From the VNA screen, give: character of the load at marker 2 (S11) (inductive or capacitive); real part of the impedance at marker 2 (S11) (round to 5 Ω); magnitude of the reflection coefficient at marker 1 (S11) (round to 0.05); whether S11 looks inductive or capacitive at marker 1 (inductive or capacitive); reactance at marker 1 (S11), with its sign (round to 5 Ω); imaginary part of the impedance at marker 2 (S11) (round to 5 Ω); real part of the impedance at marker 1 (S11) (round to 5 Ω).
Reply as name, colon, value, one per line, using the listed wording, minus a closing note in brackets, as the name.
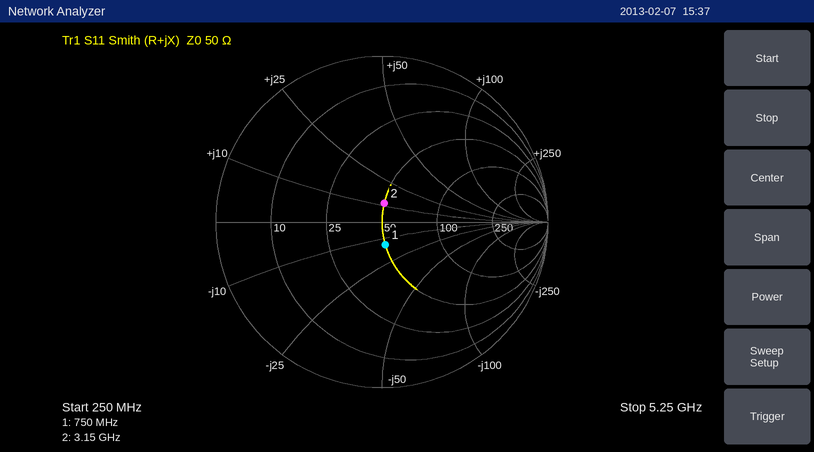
character of the load at marker 2 (S11): inductive
real part of the impedance at marker 2 (S11): 50 Ω
magnitude of the reflection coefficient at marker 1 (S11): 0.15
whether S11 looks inductive or capacitive at marker 1: capacitive
reactance at marker 1 (S11), with its sign: -15 Ω
imaginary part of the impedance at marker 2 (S11): +10 Ω
real part of the impedance at marker 1 (S11): 50 Ω
